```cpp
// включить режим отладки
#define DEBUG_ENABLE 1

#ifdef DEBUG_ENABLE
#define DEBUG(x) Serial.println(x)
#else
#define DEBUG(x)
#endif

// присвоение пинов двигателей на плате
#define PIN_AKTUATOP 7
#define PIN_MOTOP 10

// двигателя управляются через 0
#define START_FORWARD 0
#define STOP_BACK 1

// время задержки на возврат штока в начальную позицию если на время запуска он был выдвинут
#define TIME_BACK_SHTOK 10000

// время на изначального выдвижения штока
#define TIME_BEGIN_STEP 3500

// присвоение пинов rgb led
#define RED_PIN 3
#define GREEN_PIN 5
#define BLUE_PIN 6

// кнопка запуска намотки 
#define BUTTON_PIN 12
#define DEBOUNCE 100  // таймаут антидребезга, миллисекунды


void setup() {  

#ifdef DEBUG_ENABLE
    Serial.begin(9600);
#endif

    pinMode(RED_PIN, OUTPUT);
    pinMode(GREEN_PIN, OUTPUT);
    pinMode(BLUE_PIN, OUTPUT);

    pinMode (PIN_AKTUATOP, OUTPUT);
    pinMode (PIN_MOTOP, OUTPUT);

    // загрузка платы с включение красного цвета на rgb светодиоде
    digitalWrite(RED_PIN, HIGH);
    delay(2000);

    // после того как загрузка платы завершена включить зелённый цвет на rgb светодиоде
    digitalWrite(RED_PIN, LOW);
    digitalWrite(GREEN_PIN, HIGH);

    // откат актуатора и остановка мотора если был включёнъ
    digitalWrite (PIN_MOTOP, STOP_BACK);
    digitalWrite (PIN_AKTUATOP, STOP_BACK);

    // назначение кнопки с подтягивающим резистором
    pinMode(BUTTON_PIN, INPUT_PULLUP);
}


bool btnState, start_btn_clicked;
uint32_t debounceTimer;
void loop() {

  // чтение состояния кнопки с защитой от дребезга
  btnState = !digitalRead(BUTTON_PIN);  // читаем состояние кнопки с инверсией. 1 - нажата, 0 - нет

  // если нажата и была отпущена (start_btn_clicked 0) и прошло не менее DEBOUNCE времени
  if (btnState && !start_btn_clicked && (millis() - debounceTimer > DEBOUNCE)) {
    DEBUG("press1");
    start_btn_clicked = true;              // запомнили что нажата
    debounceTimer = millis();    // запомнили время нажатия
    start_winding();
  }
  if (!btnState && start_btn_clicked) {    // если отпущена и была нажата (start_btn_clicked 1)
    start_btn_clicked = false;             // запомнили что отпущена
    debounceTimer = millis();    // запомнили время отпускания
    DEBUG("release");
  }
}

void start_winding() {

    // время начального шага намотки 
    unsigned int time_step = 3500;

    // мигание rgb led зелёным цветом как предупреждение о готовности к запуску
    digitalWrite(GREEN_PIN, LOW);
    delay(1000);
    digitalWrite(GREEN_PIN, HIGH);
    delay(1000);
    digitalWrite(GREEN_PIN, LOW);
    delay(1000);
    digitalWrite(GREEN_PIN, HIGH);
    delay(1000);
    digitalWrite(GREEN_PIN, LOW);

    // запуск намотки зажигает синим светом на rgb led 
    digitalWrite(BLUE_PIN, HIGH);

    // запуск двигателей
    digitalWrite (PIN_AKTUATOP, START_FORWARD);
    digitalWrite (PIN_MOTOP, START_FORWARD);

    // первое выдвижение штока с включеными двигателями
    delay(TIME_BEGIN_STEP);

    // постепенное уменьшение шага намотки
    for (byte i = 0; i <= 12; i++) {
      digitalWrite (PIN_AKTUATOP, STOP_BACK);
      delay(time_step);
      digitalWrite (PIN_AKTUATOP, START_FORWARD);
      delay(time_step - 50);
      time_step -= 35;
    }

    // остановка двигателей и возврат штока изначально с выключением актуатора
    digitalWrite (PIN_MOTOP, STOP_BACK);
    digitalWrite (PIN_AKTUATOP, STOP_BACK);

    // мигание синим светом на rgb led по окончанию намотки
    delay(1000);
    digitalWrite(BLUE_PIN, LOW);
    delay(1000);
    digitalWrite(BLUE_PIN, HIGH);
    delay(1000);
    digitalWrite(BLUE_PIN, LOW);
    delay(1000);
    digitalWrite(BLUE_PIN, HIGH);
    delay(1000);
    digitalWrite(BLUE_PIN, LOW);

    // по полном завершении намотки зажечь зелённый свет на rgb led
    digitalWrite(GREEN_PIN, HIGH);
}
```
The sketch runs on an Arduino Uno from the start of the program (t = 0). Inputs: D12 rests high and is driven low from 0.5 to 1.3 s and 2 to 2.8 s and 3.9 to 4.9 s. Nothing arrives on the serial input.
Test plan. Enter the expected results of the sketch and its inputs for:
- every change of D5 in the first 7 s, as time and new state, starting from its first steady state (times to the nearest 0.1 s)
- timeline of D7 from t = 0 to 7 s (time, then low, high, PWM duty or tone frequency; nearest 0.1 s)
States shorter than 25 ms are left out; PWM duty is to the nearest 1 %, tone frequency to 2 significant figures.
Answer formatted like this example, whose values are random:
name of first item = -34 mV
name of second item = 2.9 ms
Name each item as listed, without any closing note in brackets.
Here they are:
every change of D5 in the first 7 s, as time and new state, starting from its first steady state = 0 s low; 3 s high; 4 s low; 5 s high; 6 s low
timeline of D7 from t = 0 to 7 s = 0 s low; 2 s high; 6 s low
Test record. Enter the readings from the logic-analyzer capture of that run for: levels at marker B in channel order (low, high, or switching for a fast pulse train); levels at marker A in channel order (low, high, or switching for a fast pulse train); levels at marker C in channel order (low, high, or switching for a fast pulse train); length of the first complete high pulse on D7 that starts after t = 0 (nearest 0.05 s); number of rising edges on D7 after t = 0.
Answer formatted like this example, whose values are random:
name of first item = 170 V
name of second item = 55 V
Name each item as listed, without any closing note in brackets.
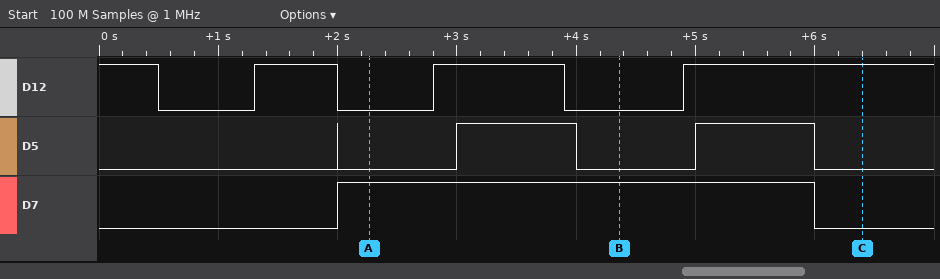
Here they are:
levels at marker B in channel order = D12 low, D5 low, D7 high
levels at marker A in channel order = D12 low, D5 low, D7 high
levels at marker C in channel order = D12 high, D5 low, D7 low
length of the first complete high pulse on D7 that starts after t = 0 = 4.00 s
number of rising edges on D7 after t = 0 = 1
